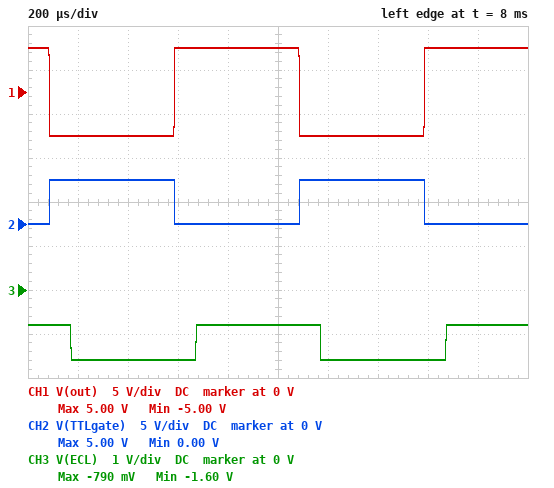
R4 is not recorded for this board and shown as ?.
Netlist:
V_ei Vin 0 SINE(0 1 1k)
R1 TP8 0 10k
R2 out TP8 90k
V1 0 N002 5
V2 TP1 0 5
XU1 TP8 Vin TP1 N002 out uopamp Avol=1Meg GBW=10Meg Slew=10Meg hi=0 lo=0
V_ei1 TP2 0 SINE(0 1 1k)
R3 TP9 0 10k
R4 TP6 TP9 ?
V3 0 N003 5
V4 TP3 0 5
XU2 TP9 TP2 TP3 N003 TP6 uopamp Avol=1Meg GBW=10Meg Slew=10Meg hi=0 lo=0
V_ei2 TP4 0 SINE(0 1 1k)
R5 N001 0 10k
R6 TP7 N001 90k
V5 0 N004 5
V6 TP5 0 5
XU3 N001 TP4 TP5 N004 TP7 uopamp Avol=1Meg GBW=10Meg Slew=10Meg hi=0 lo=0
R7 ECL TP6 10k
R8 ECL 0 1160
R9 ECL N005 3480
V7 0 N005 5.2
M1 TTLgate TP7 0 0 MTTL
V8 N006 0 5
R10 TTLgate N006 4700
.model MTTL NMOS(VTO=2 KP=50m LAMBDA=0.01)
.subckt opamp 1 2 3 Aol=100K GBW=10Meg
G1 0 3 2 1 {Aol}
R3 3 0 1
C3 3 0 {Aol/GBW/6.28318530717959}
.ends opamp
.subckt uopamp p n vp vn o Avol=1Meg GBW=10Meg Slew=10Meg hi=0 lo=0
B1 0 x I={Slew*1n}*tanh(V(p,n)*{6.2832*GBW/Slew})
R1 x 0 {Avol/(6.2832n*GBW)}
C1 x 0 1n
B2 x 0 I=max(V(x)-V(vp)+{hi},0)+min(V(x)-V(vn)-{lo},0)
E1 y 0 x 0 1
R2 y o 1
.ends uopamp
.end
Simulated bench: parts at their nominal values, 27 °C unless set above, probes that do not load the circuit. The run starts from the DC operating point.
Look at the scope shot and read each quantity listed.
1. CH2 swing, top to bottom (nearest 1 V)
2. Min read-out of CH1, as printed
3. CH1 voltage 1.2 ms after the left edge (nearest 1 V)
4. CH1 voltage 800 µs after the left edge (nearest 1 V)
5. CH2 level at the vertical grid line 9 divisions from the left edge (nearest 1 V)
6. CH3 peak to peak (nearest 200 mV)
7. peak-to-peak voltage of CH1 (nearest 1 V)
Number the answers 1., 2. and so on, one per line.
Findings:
1. 5 V
2. -5.00 V
3. -5 V
4. 5 V
5. 0 V
6. 800 mV
7. 10 V
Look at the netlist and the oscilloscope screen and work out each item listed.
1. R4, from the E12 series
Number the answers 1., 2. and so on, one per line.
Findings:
1. 47 kΩ
